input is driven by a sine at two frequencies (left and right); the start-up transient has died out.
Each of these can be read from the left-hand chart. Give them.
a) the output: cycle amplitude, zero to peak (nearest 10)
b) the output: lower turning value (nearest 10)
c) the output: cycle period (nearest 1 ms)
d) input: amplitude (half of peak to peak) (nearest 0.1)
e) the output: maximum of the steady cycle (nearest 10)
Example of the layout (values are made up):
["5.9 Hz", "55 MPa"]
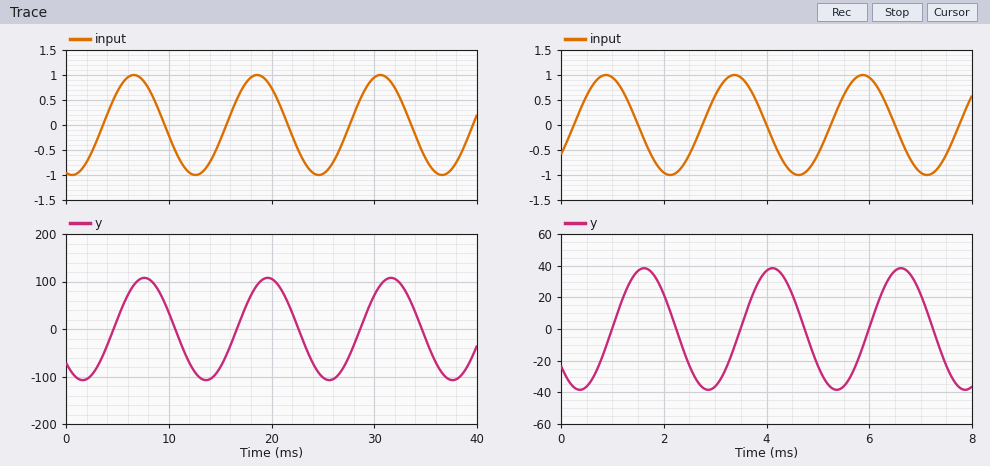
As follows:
["110", "-110", "12 ms", "1.0", "110"]
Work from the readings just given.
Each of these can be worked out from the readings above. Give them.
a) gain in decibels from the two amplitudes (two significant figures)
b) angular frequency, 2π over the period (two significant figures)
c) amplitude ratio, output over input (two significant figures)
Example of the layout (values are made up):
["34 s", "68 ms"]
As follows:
["41 dB", "0.52 rad/ms", "110"]
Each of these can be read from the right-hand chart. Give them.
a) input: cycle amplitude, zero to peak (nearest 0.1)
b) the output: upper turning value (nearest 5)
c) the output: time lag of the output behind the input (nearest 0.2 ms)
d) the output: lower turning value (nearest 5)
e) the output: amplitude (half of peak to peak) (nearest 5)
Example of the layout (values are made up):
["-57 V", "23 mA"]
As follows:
["1.0", "40", "0.8 ms", "-40", "40"]
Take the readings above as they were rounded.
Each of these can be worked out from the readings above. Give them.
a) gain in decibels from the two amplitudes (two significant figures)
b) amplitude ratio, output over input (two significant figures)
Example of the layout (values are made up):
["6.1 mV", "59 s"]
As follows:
["32 dB", "40"]
